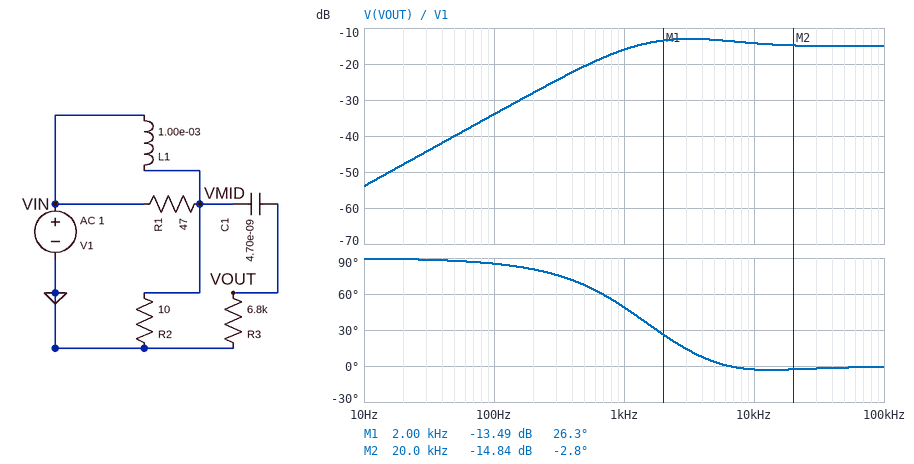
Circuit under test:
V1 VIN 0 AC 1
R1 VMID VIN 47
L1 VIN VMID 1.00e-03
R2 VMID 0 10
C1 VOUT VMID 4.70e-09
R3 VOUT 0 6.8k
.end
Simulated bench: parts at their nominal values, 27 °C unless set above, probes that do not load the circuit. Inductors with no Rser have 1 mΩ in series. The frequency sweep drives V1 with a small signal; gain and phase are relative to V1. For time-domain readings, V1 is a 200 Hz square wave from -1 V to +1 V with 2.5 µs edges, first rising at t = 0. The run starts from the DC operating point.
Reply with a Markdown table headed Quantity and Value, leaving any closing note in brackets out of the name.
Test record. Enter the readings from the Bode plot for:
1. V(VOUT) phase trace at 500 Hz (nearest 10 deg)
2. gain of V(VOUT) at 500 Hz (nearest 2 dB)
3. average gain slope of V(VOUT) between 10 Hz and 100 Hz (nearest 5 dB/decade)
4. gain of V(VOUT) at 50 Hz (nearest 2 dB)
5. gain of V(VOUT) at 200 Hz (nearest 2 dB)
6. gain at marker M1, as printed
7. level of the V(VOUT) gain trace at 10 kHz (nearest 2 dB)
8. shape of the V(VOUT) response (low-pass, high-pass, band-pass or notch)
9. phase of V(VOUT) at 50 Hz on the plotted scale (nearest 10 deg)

| Quantity | Value |
|---|---|
| V(VOUT) phase trace at 500 Hz | 70 deg |
| gain of V(VOUT) at 500 Hz | -20 dB |
| average gain slope of V(VOUT) between 10 Hz and 100 Hz | 20 dB/decade |
| gain of V(VOUT) at 50 Hz | -40 dB |
| gain of V(VOUT) at 200 Hz | -28 dB |
| gain at marker M1, as printed | -13.49 dB |
| level of the V(VOUT) gain trace at 10 kHz | -14 dB |
| shape of the V(VOUT) response | high-pass |
| phase of V(VOUT) at 50 Hz on the plotted scale | 90 deg |
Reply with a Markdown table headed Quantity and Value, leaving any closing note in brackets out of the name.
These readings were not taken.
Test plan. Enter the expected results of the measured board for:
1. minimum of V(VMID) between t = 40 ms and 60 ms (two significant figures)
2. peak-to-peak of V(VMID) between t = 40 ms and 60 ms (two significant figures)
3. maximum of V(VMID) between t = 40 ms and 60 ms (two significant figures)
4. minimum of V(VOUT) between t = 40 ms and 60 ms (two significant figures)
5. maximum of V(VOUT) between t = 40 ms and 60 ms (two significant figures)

| Quantity | Value |
|---|---|
| minimum of V(VMID) between t = 40 ms and 60 ms | -1.0 V |
| peak-to-peak of V(VMID) between t = 40 ms and 60 ms | 2.0 V |
| maximum of V(VMID) between t = 40 ms and 60 ms | 1.0 V |
| minimum of V(VOUT) between t = 40 ms and 60 ms | -370 mV |
| maximum of V(VOUT) between t = 40 ms and 60 ms | 370 mV |
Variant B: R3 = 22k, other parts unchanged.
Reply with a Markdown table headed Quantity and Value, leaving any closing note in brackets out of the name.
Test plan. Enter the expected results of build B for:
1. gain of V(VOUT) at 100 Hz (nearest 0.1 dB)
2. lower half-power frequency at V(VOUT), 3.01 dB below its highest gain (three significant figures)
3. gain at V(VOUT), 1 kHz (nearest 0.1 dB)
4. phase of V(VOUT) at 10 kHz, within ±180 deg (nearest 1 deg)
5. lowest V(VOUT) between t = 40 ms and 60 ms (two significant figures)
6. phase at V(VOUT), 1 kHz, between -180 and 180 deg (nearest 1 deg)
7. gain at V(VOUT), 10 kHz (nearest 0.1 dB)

| Quantity | Value |
|---|---|
| gain of V(VOUT) at 100 Hz | -23.8 dB |
| lower half-power frequency at V(VOUT), 3.01 dB below its highest gain | 600 Hz |
| gain at V(VOUT), 1 kHz | -7.2 dB |
| phase of V(VOUT) at 10 kHz, within ±180 deg | -21 deg |
| lowest V(VOUT) between t = 40 ms and 60 ms | -700 mV |
| phase at V(VOUT), 1 kHz, between -180 and 180 deg | 27 deg |
| gain at V(VOUT), 10 kHz | -13.4 dB |
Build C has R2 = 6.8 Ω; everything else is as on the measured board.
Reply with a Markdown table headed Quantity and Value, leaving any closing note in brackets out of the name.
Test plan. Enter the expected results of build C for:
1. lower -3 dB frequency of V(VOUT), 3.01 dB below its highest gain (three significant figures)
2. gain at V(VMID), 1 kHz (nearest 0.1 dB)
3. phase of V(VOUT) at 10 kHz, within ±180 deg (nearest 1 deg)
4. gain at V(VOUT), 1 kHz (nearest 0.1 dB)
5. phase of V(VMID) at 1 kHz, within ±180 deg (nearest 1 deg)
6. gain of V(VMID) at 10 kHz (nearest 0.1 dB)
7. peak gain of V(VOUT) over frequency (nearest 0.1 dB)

| Quantity | Value |
|---|---|
| lower -3 dB frequency of V(VOUT), 3.01 dB below its highest gain | 762 Hz |
| gain at V(VMID), 1 kHz | -3.2 dB |
| phase of V(VOUT) at 10 kHz, within ±180 deg | -5 deg |
| gain at V(VOUT), 1 kHz | -17.3 dB |
| phase of V(VMID) at 1 kHz, within ±180 deg | -39 deg |
| gain of V(VMID) at 10 kHz | -16.1 dB |
| peak gain of V(VOUT) over frequency | -15.5 dB |
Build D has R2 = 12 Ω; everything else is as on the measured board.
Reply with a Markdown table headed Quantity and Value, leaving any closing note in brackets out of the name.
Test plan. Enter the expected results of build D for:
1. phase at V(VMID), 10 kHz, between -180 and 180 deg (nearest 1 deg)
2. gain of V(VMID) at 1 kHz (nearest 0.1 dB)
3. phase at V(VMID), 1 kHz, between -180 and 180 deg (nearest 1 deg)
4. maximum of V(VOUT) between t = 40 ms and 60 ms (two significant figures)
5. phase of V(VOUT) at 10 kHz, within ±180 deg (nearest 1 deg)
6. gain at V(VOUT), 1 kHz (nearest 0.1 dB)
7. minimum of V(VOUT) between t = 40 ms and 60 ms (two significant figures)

| Quantity | Value |
|---|---|
| phase at V(VMID), 10 kHz, between -180 and 180 deg | -28 deg |
| gain of V(VMID) at 1 kHz | -1.5 dB |
| phase at V(VMID), 1 kHz, between -180 and 180 deg | -26 deg |
| maximum of V(VOUT) between t = 40 ms and 60 ms | 420 mV |
| phase of V(VOUT) at 10 kHz, within ±180 deg | -2 deg |
| gain at V(VOUT), 1 kHz | -15.6 dB |
| minimum of V(VOUT) between t = 40 ms and 60 ms | -420 mV |
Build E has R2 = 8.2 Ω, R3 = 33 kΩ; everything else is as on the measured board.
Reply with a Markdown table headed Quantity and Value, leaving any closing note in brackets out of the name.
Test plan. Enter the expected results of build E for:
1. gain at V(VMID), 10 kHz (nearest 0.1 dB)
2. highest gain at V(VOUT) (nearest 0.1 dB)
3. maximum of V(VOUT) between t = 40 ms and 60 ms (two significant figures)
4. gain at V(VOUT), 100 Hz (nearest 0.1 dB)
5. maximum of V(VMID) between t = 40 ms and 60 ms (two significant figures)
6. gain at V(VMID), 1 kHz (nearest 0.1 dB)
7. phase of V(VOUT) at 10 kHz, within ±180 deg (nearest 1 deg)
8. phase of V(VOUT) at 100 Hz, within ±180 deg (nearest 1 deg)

| Quantity | Value |
|---|---|
| gain at V(VMID), 10 kHz | -14.7 dB |
| highest gain at V(VOUT) | -5.6 dB |
| maximum of V(VOUT) between t = 40 ms and 60 ms | 780 mV |
| gain at V(VOUT), 100 Hz | -20.3 dB |
| maximum of V(VMID) between t = 40 ms and 60 ms | 1.0 V |
| gain at V(VMID), 1 kHz | -2.5 dB |
| phase of V(VOUT) at 10 kHz, within ±180 deg | -25 deg |
| phase of V(VOUT) at 100 Hz, within ±180 deg | 80 deg |
